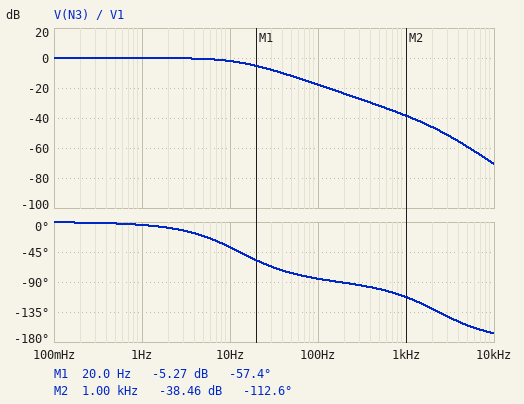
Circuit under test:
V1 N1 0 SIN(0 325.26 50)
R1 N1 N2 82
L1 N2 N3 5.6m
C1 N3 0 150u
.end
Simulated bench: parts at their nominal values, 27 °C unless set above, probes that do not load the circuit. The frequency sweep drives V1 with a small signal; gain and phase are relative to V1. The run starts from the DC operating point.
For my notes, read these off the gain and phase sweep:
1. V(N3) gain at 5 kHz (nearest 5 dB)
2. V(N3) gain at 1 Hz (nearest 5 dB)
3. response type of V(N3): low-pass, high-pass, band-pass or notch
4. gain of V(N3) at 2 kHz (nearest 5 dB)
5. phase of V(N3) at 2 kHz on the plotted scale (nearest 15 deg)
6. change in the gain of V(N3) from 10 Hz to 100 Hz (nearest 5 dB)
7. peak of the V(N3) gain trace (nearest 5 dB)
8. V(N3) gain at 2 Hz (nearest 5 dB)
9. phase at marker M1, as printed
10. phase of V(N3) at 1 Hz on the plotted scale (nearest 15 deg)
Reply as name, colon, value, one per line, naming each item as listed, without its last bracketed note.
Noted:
V(N3) gain at 5 kHz: -60 dB
V(N3) gain at 1 Hz: 0 dB
response type of V(N3): low-pass, high-pass, band-pass or notch: low-pass
gain of V(N3) at 2 kHz: -45 dB
phase of V(N3) at 2 kHz on the plotted scale: -135 deg
change in the gain of V(N3) from 10 Hz to 100 Hz: -15 dB
peak of the V(N3) gain trace: 0 dB
V(N3) gain at 2 Hz: 0 dB
phase at marker M1, as printed: -57.4 deg
phase of V(N3) at 1 Hz on the plotted scale: 0 deg
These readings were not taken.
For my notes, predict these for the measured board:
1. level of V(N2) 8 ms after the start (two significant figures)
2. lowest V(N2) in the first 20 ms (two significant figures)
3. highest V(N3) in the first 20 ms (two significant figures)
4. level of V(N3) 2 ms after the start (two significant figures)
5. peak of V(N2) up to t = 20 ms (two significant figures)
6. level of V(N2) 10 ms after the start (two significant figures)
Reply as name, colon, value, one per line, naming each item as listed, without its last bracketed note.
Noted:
level of V(N2) 8 ms after the start: 110 V
lowest V(N2) in the first 20 ms: -59 V
highest V(N3) in the first 20 ms: 120 V
level of V(N3) 2 ms after the start: 14 V
peak of V(N2) up to t = 20 ms: 110 V
level of V(N2) 10 ms after the start: 110 V
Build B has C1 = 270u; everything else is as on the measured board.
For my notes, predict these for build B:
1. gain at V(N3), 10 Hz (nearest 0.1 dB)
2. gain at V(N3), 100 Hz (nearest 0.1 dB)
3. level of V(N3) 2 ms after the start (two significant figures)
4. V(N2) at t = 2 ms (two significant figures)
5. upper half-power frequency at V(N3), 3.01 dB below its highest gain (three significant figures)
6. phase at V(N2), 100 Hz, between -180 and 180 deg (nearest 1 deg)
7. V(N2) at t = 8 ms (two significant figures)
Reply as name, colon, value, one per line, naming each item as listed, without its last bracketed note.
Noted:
gain at V(N3), 10 Hz: -4.7 dB
gain at V(N3), 100 Hz: -22.9 dB
level of V(N3) 2 ms after the start: 8.1 V
V(N2) at t = 2 ms: 13 V
upper half-power frequency at V(N3), 3.01 dB below its highest gain: 7.21 Hz
phase at V(N2), 100 Hz, between -180 and 180 deg: -88 deg
V(N2) at t = 8 ms: 67 V
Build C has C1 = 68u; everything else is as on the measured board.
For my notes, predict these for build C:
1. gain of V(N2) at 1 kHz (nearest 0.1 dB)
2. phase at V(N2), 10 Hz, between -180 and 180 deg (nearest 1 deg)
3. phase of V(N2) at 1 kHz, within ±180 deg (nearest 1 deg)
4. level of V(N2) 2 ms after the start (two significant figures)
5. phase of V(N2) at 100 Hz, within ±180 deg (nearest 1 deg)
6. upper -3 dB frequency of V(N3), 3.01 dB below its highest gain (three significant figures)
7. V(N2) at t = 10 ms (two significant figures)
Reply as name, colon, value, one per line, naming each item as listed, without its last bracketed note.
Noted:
gain of V(N2) at 1 kHz: -8.6 dB
phase at V(N2), 10 Hz, between -180 and 180 deg: -19 deg
phase of V(N2) at 1 kHz, within ±180 deg: 68 deg
level of V(N2) 2 ms after the start: 34 V
phase of V(N2) at 100 Hz, within ±180 deg: -76 deg
upper -3 dB frequency of V(N3), 3.01 dB below its highest gain: 28.9 Hz
V(N2) at t = 10 ms: 160 V
